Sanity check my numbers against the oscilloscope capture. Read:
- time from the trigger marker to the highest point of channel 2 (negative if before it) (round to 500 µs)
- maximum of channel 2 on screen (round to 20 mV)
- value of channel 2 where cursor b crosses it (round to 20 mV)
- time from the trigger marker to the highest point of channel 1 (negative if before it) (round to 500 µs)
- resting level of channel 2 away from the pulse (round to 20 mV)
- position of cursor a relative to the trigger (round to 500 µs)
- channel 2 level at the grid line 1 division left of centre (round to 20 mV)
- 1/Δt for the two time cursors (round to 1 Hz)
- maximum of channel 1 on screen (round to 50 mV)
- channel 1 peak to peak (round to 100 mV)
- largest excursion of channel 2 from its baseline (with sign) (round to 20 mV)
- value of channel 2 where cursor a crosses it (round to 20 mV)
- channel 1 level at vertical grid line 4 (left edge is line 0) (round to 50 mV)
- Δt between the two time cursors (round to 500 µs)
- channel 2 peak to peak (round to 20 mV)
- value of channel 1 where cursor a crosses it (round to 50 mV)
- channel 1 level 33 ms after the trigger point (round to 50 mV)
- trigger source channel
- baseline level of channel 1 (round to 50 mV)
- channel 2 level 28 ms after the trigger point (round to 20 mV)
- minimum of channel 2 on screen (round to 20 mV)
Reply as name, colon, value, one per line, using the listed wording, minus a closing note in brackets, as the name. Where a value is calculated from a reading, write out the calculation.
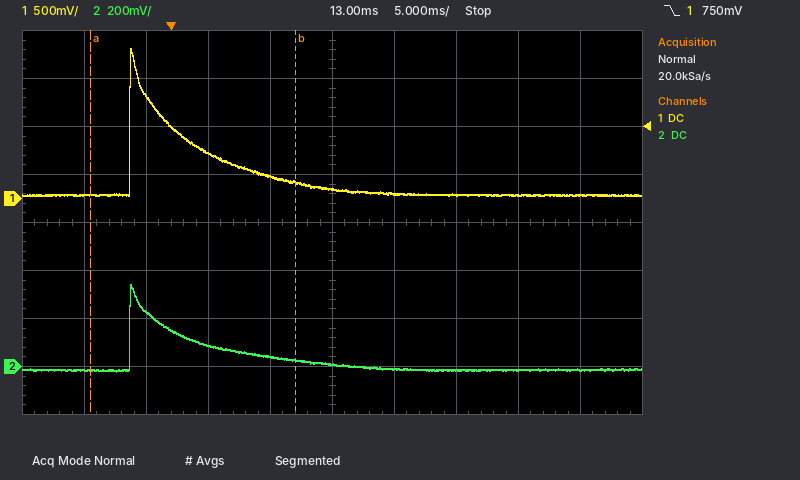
time from the trigger marker to the highest point of channel 2 (negative if before it): -3.0 ms
maximum of channel 2 on screen: 340 mV
value of channel 2 where cursor b crosses it: 20 mV
time from the trigger marker to the highest point of channel 1 (negative if before it): -3.0 ms
resting level of channel 2 away from the pulse: -20 mV
position of cursor a relative to the trigger: -6.5 ms
channel 2 level at the grid line 1 division left of centre: 40 mV
1/Δt for the two time cursors: 1 / 16.5 ms ≈ 61 Hz
maximum of channel 1 on screen: 1.55 V
channel 1 peak to peak: 1.50 V
largest excursion of channel 2 from its baseline (with sign): 340 mV − (-20 mV) = +360 mV
value of channel 2 where cursor a crosses it: -20 mV
channel 1 level at vertical grid line 4 (left edge is line 0): 250 mV
Δt between the two time cursors: 16.5 ms
channel 2 peak to peak: 340 mV − (-20 mV) = 360 mV
value of channel 1 where cursor a crosses it: 50 mV
channel 1 level 33 ms after the trigger point: 50 mV
trigger source channel: channel 1
baseline level of channel 1: 50 mV
channel 2 level 28 ms after the trigger point: -20 mV
minimum of channel 2 on screen: -20 mV
